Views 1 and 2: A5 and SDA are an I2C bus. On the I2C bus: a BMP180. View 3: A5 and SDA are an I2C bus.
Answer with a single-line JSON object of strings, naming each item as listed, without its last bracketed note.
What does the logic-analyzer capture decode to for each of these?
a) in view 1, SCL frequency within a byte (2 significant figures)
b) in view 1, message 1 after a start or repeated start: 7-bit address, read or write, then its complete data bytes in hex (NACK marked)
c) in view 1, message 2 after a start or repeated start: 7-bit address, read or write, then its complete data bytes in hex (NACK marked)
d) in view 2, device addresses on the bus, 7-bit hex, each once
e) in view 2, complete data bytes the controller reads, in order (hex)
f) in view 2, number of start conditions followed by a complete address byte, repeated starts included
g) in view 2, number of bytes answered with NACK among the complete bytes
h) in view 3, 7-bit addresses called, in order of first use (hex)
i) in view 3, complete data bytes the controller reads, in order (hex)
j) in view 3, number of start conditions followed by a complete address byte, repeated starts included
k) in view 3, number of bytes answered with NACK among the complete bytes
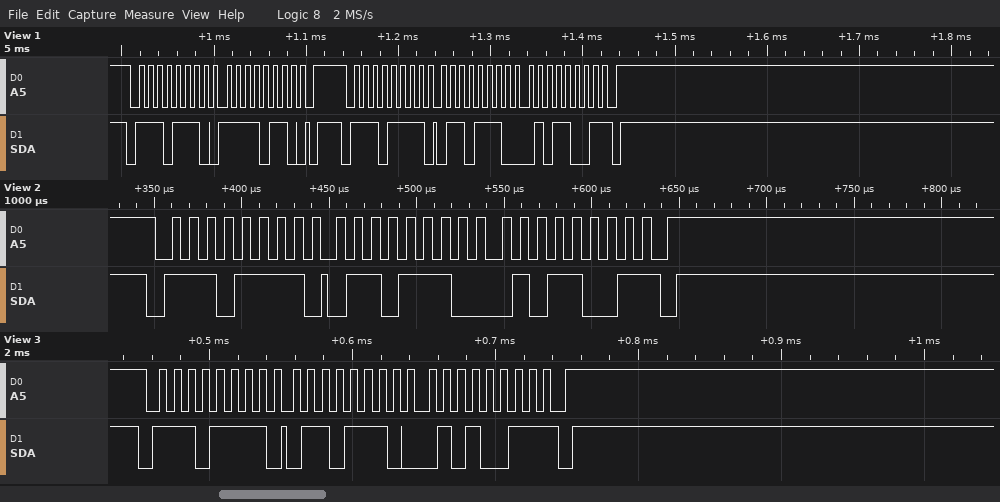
{"in view 1, SCL frequency within a byte": "100 kHz", "in view 1, message 1 after a start or repeated start: 7-bit address, read or write, then its complete data bytes in hex": "0x77 write: F6", "in view 1, message 2 after a start or repeated start: 7-bit address, read or write, then its complete data bytes in hex": "0x77 read: 6E 59 NACK", "in view 2, device addresses on the bus, 7-bit hex, each once": "0x77", "in view 2, complete data bytes the controller reads, in order": "6E 59", "in view 2, number of start conditions followed by a complete address byte, repeated starts included": "1", "in view 2, number of bytes answered with NACK among the complete bytes": "1", "in view 3, 7-bit addresses called, in order of first use": "0x77", "in view 3, complete data bytes the controller reads, in order": "6E 53", "in view 3, number of start conditions followed by a complete address byte, repeated starts included": "1", "in view 3, number of bytes answered with NACK among the complete bytes": "1"}
